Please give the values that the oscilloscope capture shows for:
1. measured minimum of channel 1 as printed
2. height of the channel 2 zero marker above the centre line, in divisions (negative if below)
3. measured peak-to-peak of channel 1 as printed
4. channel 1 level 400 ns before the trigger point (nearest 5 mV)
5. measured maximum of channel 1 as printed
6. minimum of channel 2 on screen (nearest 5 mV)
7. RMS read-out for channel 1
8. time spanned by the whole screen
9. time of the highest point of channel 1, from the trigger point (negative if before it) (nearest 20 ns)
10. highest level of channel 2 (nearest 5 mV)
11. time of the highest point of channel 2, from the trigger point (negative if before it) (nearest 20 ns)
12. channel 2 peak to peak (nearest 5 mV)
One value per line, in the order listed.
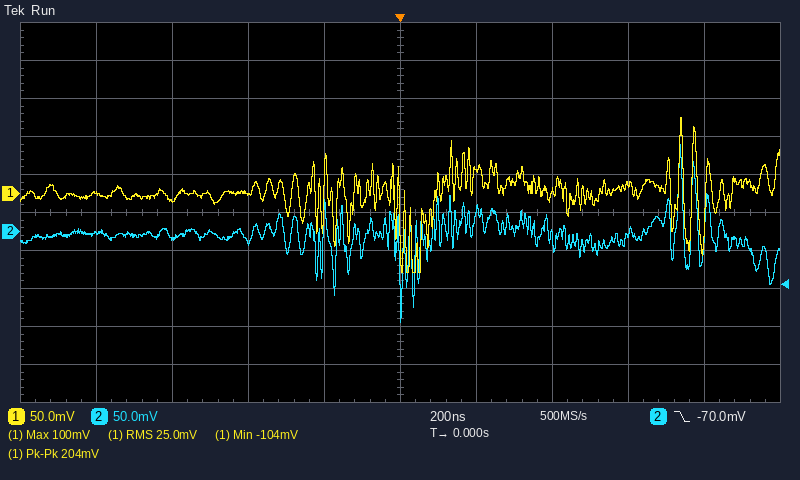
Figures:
-104 mV
-0.5 div
204 mV
0 mV
100 mV
-120 mV
25.0 mV
2 µs
+740 ns
115 mV
+740 ns
235 mV
